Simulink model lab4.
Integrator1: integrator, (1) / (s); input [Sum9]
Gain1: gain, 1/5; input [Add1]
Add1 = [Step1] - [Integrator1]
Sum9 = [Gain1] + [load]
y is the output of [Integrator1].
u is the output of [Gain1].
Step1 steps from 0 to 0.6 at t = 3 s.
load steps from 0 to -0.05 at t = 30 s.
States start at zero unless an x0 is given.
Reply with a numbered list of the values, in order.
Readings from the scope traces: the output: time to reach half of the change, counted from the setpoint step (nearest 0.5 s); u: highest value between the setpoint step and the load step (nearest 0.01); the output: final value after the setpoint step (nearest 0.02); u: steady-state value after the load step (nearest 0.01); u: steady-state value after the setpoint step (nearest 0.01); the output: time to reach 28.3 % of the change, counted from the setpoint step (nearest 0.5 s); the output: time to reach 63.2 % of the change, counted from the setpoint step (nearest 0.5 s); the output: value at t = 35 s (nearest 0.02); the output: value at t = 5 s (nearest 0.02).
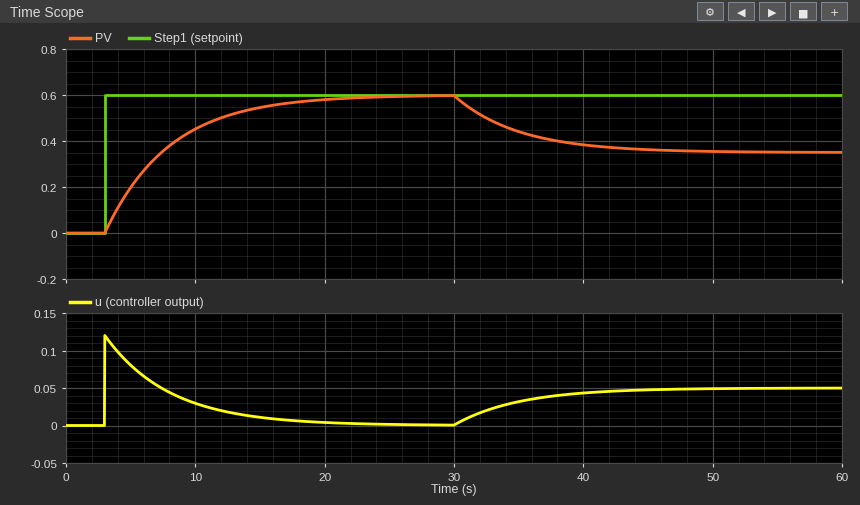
1. 3.5 s
2. 0.12
3. 0.60
4. 0.05
5. 0.00
6. 1.5 s
7. 5.0 s
8. 0.44
9. 0.20
